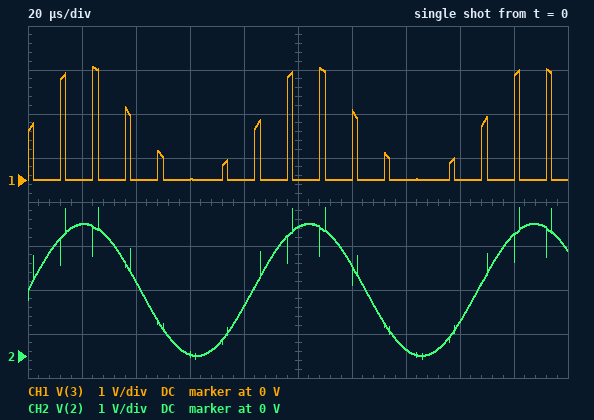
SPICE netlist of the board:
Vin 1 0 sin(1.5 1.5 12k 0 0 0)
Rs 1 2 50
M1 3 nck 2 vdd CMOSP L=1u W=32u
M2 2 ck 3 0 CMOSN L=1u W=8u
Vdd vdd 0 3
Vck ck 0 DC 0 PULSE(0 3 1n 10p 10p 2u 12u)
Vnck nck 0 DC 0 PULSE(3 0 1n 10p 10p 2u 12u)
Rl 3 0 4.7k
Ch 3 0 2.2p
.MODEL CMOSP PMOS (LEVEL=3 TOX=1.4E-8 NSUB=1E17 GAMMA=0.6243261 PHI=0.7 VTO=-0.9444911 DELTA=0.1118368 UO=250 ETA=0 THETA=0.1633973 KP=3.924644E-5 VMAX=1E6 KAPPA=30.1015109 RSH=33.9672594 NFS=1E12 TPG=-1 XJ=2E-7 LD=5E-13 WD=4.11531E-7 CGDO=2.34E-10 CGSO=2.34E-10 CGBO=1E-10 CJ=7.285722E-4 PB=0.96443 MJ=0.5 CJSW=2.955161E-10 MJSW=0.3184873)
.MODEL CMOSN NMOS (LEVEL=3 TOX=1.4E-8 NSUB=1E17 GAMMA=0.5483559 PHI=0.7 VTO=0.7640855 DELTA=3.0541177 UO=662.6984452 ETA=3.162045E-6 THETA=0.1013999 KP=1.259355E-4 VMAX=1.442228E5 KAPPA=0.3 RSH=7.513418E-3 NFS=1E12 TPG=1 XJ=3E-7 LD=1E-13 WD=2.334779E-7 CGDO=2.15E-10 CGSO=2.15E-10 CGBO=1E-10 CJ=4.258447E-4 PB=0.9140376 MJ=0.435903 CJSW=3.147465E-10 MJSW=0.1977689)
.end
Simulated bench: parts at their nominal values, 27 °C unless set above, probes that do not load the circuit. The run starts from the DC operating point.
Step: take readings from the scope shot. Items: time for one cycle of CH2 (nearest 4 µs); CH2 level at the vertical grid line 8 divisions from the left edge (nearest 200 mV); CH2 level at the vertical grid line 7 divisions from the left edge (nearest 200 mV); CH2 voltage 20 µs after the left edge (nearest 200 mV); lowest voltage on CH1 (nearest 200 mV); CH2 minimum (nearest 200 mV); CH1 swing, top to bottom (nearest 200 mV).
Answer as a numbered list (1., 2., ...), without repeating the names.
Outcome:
1. 84 µs
2. 800 mV
3. 200 mV
4. 3.0 V
5. 0 V
6. 0 V
7. 2.6 V
